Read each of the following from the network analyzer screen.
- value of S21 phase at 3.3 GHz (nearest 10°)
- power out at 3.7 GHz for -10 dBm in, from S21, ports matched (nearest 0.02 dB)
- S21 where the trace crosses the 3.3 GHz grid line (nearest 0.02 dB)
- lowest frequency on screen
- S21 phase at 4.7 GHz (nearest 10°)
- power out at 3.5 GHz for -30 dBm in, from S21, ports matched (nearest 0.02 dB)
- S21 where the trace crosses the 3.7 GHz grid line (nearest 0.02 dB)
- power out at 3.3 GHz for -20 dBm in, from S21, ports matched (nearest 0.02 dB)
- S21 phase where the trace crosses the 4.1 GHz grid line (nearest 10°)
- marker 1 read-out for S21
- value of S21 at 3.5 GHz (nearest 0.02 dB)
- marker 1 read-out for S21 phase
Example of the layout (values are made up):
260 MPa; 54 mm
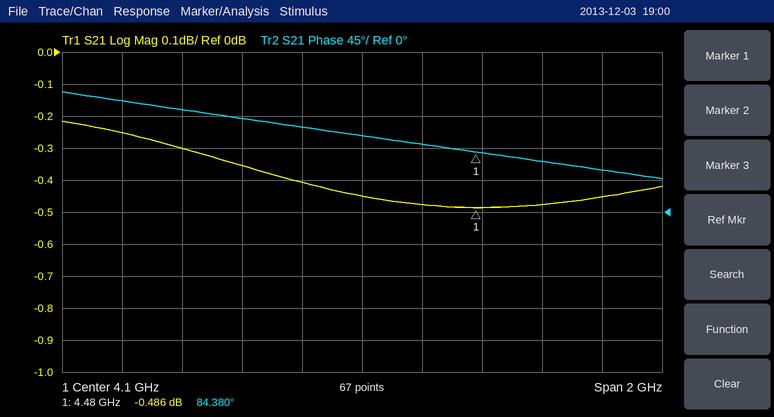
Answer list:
160°; -10.36 dBm; -0.26 dB; 3.1 GHz; 70°; -30.30 dBm; -0.36 dB; -20.26 dBm; 110°; -0.486 dB; -0.30 dB; 84.380°
